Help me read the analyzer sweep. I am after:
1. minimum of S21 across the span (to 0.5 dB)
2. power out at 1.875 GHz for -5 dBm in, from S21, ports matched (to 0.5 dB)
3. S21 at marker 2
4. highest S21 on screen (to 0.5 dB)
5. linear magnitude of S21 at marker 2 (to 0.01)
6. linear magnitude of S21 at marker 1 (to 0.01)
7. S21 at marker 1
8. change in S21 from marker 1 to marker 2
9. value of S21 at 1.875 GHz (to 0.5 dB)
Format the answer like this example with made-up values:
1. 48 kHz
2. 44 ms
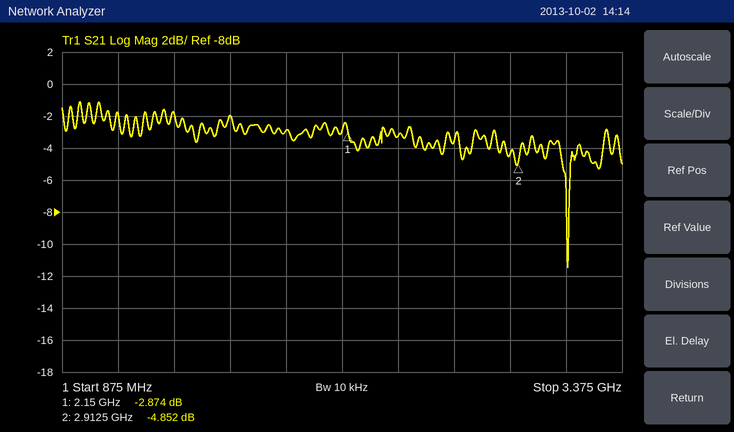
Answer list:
1. -11.5 dB
2. -8.0 dBm
3. -4.852 dB
4. -1.0 dB
5. 0.57
6. 0.72
7. -2.874 dB
8. -1.978 dB
9. -3.0 dB
